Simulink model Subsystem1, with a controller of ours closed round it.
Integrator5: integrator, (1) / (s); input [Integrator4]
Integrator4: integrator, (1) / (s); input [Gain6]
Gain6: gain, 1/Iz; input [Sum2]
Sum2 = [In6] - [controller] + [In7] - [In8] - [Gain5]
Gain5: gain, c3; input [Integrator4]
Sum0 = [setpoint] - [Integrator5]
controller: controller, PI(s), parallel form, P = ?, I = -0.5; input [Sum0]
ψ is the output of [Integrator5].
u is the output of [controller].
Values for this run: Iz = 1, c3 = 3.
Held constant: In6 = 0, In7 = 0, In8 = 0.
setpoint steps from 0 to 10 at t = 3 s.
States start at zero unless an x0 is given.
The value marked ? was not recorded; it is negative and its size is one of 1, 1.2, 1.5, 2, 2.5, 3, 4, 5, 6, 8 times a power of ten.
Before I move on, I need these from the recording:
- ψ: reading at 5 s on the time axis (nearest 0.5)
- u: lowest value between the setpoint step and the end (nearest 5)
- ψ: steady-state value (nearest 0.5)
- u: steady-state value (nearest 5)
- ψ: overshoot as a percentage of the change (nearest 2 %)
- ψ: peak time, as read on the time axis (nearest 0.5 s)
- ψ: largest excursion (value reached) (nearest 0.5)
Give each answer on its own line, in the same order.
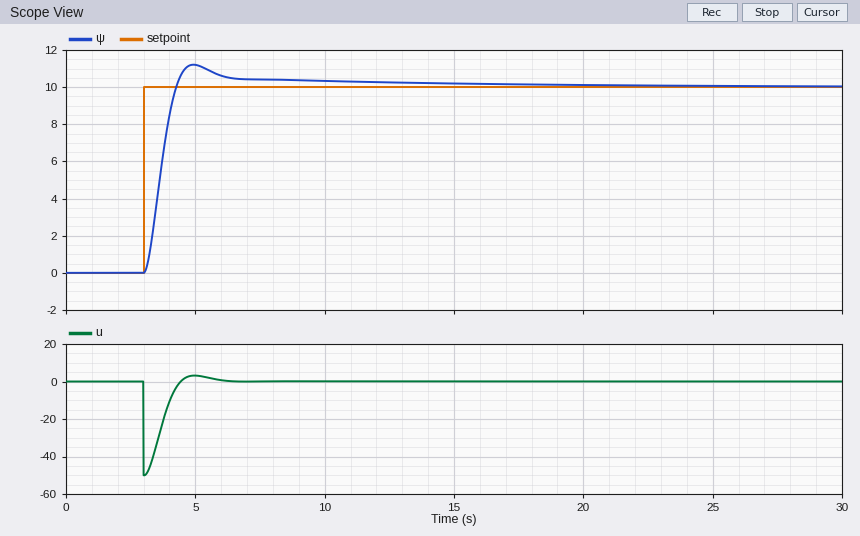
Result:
11.0
-50
10.0
0
12 %
5.0 s
11.0
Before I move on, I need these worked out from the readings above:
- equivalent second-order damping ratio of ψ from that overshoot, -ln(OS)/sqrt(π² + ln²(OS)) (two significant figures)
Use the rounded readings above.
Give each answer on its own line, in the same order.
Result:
0.56
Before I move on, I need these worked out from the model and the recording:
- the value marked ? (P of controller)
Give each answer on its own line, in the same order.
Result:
-5
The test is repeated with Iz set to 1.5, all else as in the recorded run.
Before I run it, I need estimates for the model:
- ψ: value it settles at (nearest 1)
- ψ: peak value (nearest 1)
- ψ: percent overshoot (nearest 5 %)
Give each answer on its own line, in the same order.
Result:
10
12
20 %
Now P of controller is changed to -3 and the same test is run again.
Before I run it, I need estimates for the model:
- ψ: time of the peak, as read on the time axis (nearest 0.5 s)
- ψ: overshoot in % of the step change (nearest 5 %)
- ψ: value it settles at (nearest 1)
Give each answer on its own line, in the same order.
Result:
6.5 s
15 %
10
